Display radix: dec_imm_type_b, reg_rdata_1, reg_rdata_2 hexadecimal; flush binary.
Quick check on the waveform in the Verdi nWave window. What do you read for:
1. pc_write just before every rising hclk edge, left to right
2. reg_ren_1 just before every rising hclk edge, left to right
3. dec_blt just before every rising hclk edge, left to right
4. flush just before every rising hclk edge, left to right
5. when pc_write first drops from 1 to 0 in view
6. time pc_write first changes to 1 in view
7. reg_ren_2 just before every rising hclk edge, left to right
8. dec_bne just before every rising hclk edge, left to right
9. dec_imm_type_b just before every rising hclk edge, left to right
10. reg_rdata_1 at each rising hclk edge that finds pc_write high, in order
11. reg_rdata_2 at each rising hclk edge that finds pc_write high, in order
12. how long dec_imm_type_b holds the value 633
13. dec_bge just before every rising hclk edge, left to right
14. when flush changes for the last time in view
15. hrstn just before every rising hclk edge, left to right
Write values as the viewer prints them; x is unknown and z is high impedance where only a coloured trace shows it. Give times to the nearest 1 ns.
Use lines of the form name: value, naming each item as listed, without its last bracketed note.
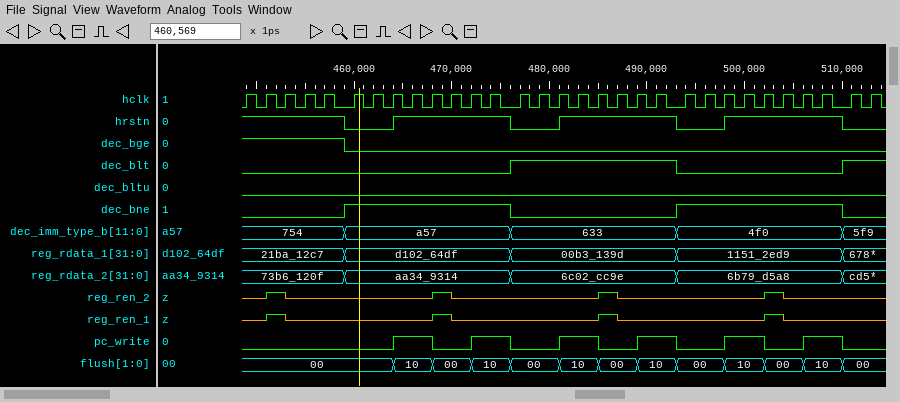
pc_write just before every rising hclk edge, left to right: 0 0 0 0 0 0 0 0 1 1 0 0 1 0 0 0 1 1 0 0 1 0 0 0 1 1 0 0 1 0 0
reg_ren_1 just before every rising hclk edge, left to right: z z 1 z z z z z z z 1 z z z z z z z 1 z z z z z z z 1 z z z z
dec_blt just before every rising hclk edge, left to right: 0 0 0 0 0 0 0 0 0 0 0 0 0 1 1 1 1 1 1 1 1 0 0 0 0 0 0 0 0 1 1
flush just before every rising hclk edge, left to right: 00, 00, 00, 00, 00, 00, 00, 00, 10, 10, 00, 00, 10, 00, 00, 00, 10, 10, 00, 00, 10, 00, 00, 00, 10, 10, 00, 00, 10, 00, 00
when pc_write first drops from 1 to 0 in view: 468 ns
time pc_write first changes to 1 in view: 464 ns
reg_ren_2 just before every rising hclk edge, left to right: z z 1 z z z z z z z 1 z z z z z z z 1 z z z z z z z 1 z z z z
dec_bne just before every rising hclk edge, left to right: 0 0 0 0 0 1 1 1 1 1 1 1 1 0 0 0 0 0 0 0 0 1 1 1 1 1 1 1 1 0 0
dec_imm_type_b just before every rising hclk edge, left to right: 754, 754, 754, 754, 754, a57, a57, a57, a57, a57, a57, a57, a57, 633, 633, 633, 633, 633, 633, 633, 633, 4f0, 4f0, 4f0, 4f0, 4f0, 4f0, 4f0, 4f0, 5f9, 5f9
reg_rdata_1 at each rising hclk edge that finds pc_write high, in order: d102_64df, d102_64df, d102_64df, 00b3_139d, 00b3_139d, 00b3_139d, 1151_2ed9, 1151_2ed9, 1151_2ed9
reg_rdata_2 at each rising hclk edge that finds pc_write high, in order: aa34_9314, aa34_9314, aa34_9314, 6c02_cc9e, 6c02_cc9e, 6c02_cc9e, 6b79_d5a8, 6b79_d5a8, 6b79_d5a8
how long dec_imm_type_b holds the value 633: 17 ns
dec_bge just before every rising hclk edge, left to right: 1 1 1 1 1 0 0 0 0 0 0 0 0 0 0 0 0 0 0 0 0 0 0 0 0 0 0 0 0 0 0
when flush changes for the last time in view: 510 ns
hrstn just before every rising hclk edge, left to right: 1 1 1 1 1 0 0 0 1 1 1 1 1 0 0 0 1 1 1 1 1 0 0 0 1 1 1 1 1 0 0
